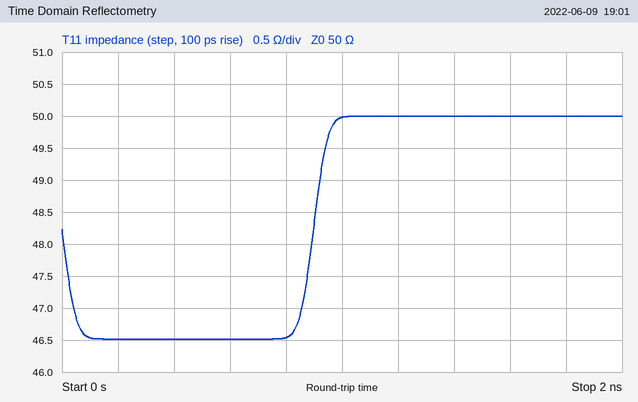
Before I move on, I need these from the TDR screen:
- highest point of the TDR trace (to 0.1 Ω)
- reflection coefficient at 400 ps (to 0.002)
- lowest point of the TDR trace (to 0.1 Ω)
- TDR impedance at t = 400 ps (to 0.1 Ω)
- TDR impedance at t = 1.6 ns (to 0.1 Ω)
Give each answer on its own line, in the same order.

50.0 Ω
-0.036
46.5 Ω
46.5 Ω
50.0 Ω
